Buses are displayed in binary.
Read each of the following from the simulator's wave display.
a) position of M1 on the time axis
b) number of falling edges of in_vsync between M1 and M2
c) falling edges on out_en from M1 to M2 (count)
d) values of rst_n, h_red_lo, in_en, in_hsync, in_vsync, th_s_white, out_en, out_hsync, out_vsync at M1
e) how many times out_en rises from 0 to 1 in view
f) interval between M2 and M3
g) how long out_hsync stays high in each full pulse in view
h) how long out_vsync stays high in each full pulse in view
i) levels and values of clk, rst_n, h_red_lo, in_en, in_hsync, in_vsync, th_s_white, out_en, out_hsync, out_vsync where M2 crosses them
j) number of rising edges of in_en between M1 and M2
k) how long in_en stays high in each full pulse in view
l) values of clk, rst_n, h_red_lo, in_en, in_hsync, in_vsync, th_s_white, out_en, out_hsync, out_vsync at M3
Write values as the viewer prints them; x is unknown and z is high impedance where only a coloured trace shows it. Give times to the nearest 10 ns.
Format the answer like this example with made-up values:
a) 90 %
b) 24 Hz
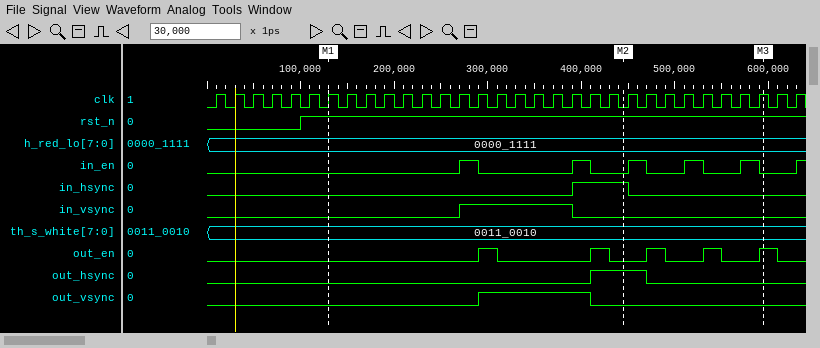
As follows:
a) 130 ns
b) 1
c) 2
d) rst_n=1, h_red_lo=0000_1111, in_en=0, in_hsync=0, in_vsync=0, th_s_white=0011_0010, out_en=0, out_hsync=0, out_vsync=0
e) 5
f) 150 ns
g) 60 ns
h) 120 ns
i) clk=0, rst_n=1, h_red_lo=0000_1111, in_en=0, in_hsync=1, in_vsync=0, th_s_white=0011_0010, out_en=0, out_hsync=1, out_vsync=0
j) 2
k) 20 ns, 20 ns, 20 ns, 20 ns, 20 ns
l) clk=1, rst_n=1, h_red_lo=0000_1111, in_en=0, in_hsync=0, in_vsync=0, th_s_white=0011_0010, out_en=1, out_hsync=0, out_vsync=0
